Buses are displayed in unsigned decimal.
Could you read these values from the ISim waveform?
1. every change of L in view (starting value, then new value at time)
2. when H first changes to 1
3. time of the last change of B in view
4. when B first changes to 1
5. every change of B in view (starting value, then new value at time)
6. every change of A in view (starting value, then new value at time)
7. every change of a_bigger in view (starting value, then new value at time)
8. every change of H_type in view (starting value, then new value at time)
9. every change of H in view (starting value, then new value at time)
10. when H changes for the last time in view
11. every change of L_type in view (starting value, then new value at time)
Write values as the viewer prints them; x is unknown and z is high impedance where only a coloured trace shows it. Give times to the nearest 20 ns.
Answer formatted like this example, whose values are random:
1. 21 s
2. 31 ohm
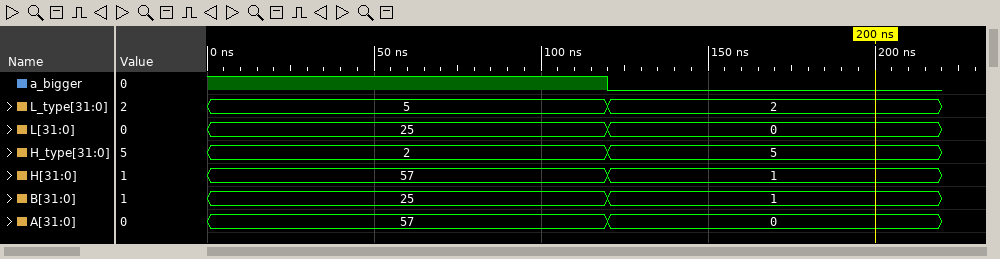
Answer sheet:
1. 25, 0 at 120 ns
2. 120 ns
3. 120 ns
4. 120 ns
5. 25, 1 at 120 ns
6. 57, 0 at 120 ns
7. 1, 0 at 120 ns
8. 2, 5 at 120 ns
9. 57, 1 at 120 ns
10. 120 ns
11. 5, 2 at 120 ns
